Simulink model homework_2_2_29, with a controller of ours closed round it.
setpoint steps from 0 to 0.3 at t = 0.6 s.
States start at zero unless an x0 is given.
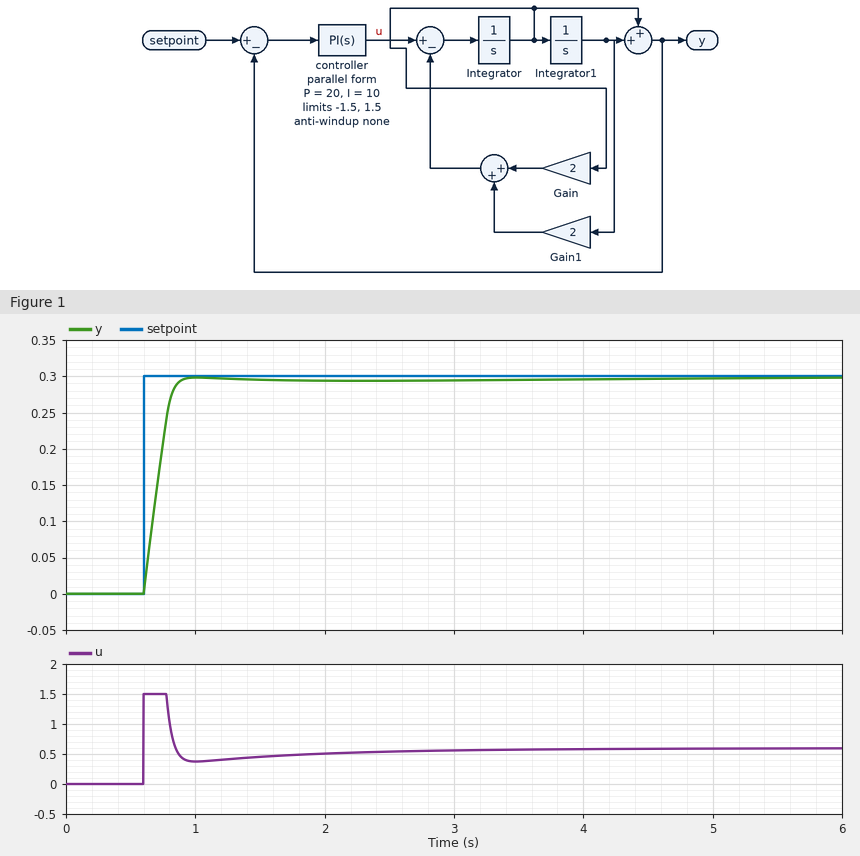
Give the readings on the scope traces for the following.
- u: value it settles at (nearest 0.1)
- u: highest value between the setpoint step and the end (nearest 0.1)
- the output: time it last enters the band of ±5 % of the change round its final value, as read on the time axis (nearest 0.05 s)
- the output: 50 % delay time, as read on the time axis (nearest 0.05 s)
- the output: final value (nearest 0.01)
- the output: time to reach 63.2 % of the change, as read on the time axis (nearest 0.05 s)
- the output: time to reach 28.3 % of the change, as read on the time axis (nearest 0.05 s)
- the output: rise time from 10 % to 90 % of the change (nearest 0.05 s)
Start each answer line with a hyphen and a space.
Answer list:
- 0.6
- 1.5
- 0.85 s
- 0.70 s
- 0.30
- 0.75 s
- 0.65 s
- 0.20 s
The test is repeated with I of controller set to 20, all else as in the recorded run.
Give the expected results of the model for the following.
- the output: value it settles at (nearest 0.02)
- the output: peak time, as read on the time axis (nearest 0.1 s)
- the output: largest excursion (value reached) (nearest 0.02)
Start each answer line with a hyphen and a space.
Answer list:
- 0.30
- 1.0 s
- 0.32
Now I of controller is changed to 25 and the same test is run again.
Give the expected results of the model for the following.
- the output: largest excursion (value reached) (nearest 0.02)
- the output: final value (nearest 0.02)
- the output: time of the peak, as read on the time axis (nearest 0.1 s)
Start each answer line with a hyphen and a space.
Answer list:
- 0.32
- 0.30
- 1.0 s
